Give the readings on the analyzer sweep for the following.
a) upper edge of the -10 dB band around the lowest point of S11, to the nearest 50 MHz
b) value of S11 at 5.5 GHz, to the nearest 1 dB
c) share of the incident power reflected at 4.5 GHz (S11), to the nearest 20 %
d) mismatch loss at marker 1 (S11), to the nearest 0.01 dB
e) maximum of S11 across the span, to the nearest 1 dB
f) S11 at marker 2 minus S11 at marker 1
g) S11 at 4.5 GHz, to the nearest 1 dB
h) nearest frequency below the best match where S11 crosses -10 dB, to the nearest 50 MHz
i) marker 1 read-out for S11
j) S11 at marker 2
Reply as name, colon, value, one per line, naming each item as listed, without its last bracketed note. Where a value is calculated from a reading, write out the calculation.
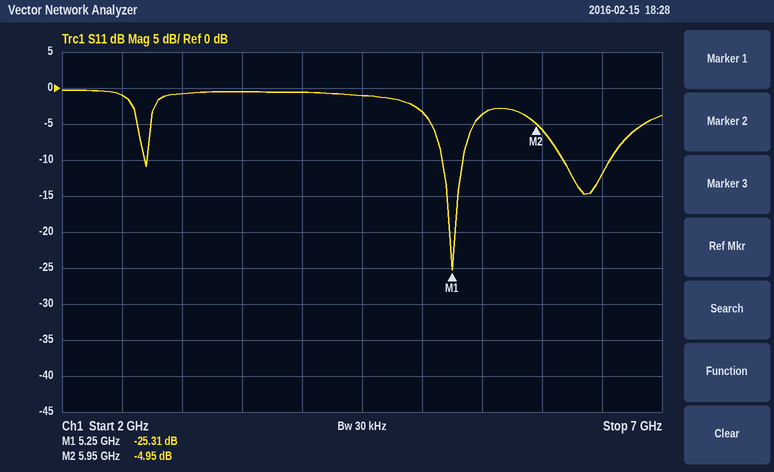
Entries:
upper edge of the -10 dB band around the lowest point of S11, to the nearest 50 MHz: 5.35 GHz
value of S11 at 5.5 GHz, to the nearest 1 dB: -4 dB
share of the incident power reflected at 4.5 GHz (S11), to the nearest 20 %: 10^(-1/10) ≈ 79.4 %, so 80 % to the nearest 20 %
mismatch loss at marker 1 (S11), to the nearest 0.01 dB: −10 log10(1 − 10^(-25.31/10)) ≈ 0.01 dB
maximum of S11 across the span, to the nearest 1 dB: 0 dB
S11 at marker 2 minus S11 at marker 1: -4.95 − (-25.31) = 20.36 dB
S11 at 4.5 GHz, to the nearest 1 dB: -1 dB
nearest frequency below the best match where S11 crosses -10 dB, to the nearest 50 MHz: 5.15 GHz
marker 1 read-out for S11: -25.31 dB
S11 at marker 2: -4.95 dB
